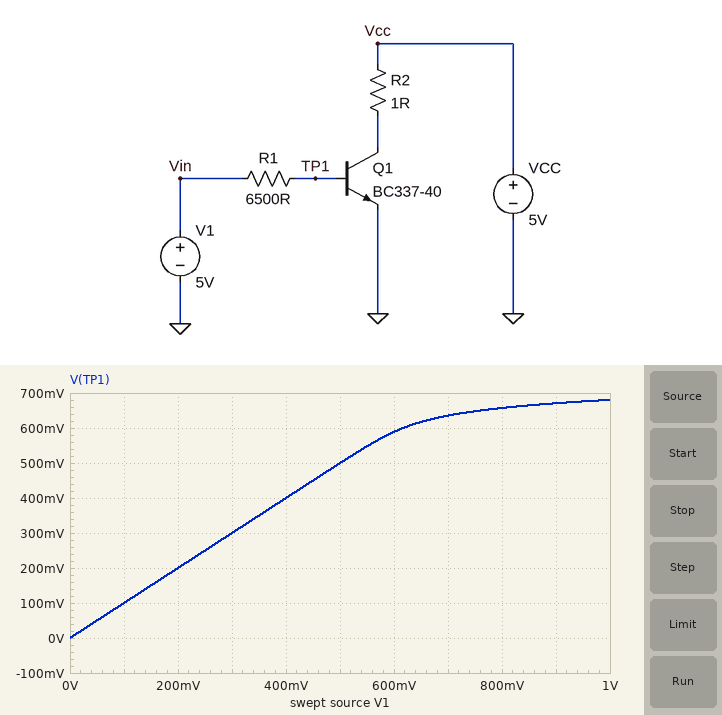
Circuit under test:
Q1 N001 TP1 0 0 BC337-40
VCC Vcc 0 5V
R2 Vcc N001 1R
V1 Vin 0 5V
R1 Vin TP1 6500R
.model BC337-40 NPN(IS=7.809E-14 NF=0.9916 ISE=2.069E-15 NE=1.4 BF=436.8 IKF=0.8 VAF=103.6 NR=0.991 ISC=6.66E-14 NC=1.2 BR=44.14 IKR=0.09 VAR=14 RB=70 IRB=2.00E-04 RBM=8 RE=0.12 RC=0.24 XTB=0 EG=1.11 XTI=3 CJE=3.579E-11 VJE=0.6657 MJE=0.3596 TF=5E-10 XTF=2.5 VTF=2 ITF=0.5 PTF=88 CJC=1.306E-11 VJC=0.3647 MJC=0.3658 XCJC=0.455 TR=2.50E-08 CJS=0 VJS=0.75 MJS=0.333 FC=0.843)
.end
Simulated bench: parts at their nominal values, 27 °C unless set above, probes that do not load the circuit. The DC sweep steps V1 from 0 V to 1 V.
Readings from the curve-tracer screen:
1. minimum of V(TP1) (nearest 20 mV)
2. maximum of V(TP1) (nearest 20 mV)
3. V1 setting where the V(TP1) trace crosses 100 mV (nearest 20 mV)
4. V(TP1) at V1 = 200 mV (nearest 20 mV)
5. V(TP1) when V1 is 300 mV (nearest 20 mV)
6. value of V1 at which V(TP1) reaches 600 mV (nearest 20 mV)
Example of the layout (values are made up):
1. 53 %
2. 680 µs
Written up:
1. 0 V
2. 680 mV
3. 100 mV
4. 200 mV
5. 300 mV
6. 620 mV
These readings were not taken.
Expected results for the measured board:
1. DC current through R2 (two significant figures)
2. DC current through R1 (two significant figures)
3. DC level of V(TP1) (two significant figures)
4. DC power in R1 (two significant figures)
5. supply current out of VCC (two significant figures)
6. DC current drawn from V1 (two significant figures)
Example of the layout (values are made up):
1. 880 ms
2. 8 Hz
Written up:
1. 220 mA
2. 650 µA
3. 790 mV
4. 2.7 mW
5. 220 mA
6. 650 µA
